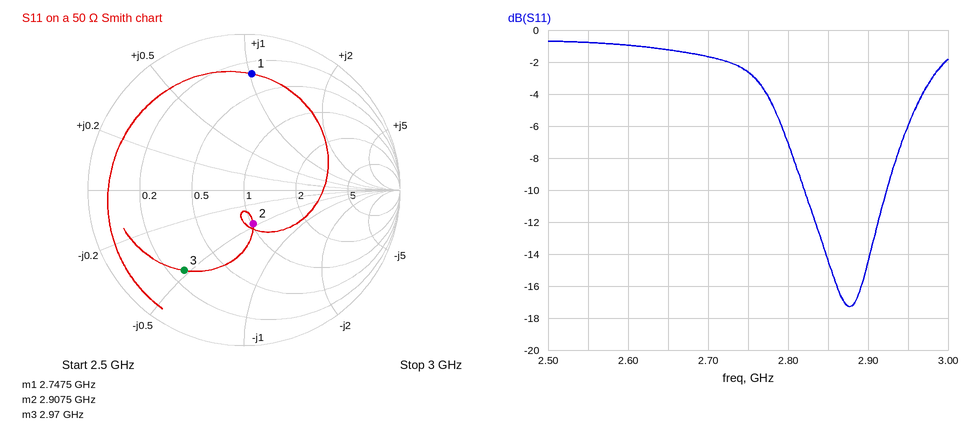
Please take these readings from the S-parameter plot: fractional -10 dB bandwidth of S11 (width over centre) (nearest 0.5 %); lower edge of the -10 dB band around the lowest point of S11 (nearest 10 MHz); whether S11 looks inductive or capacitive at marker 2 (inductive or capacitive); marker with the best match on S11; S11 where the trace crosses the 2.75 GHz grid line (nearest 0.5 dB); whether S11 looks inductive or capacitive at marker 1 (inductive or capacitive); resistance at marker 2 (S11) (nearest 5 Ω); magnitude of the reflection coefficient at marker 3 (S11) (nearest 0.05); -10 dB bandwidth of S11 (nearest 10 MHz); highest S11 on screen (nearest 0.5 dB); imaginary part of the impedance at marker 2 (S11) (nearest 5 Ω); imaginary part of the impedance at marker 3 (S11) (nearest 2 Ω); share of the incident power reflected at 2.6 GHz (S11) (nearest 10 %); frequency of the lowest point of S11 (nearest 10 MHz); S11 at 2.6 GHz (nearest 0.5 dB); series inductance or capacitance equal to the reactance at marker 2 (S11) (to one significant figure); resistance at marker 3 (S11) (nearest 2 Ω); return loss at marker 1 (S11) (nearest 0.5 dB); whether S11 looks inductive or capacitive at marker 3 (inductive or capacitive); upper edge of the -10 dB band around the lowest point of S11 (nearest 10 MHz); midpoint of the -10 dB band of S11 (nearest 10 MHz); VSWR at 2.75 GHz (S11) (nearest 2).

3.5 %
2.82 GHz
capacitive
marker 2
-2.5 dB
inductive
50 Ω
0.65
100 MHz
-0.5 dB
-25 Ω
-24 Ω
80 %
2.88 GHz
-1.0 dB
2 pF
14 Ω
2.5 dB
capacitive
2.92 GHz
2.87 GHz
6
